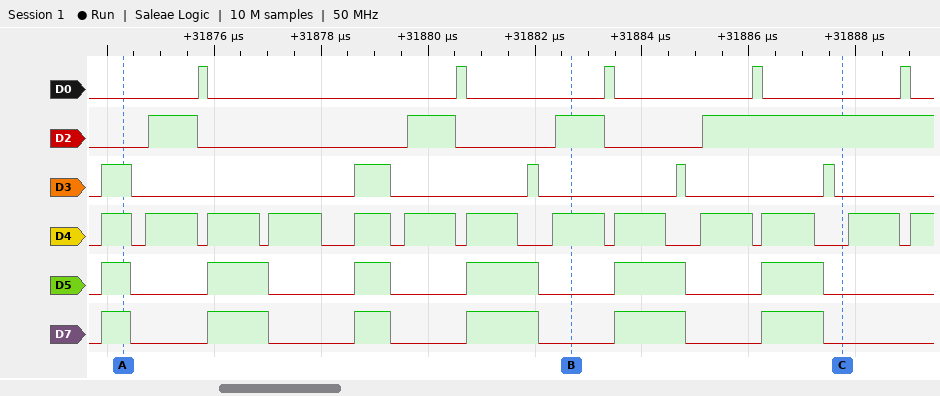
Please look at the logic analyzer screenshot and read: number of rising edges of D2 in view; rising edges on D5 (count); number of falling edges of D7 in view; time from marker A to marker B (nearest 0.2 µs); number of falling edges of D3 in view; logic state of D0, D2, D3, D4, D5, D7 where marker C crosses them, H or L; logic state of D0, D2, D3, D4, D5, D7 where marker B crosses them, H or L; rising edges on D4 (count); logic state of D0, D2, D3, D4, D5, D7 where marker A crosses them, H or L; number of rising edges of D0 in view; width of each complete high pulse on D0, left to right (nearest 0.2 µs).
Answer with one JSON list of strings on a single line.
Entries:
["4", "6", "6", "8.4 µs", "5", "D0=L, D2=H, D3=L, D4=L, D5=L, D7=L", "D0=L, D2=H, D3=L, D4=H, D5=L, D7=L", "13", "D0=L, D2=L, D3=H, D4=H, D5=H, D7=H", "5", "0.2 µs, 0.2 µs, 0.2 µs, 0.2 µs, 0.2 µs"]
